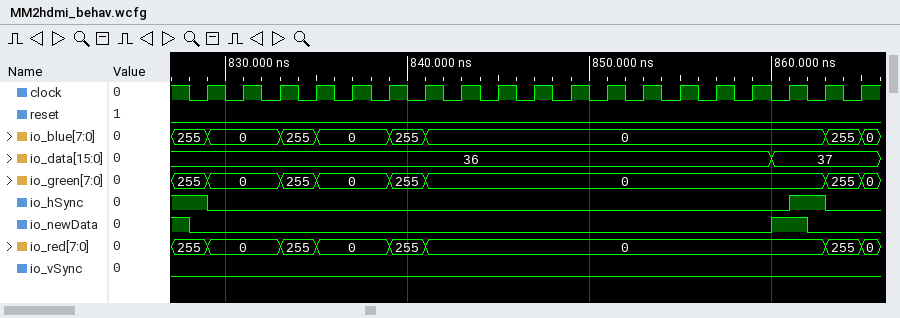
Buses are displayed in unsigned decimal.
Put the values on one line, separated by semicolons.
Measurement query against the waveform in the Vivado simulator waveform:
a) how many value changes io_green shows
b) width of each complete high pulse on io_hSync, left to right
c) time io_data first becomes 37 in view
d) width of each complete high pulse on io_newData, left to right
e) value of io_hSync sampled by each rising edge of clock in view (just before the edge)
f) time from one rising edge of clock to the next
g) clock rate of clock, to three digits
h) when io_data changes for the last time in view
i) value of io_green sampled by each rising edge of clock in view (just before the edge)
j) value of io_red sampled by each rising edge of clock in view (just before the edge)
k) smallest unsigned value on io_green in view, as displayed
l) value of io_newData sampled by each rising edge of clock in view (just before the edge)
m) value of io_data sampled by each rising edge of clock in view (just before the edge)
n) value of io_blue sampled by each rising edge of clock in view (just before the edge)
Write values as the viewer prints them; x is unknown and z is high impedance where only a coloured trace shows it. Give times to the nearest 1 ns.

7; 2 ns; 860 ns; 2 ns; 1 0 0 0 0 0 0 0 0 0 0 0 0 0 0 0 0 1 0; 2 ns; 500 MHz; 860 ns; 255, 0, 0, 255, 0, 0, 255, 0, 0, 0, 0, 0, 0, 0, 0, 0, 0, 0, 255; 255, 0, 0, 255, 0, 0, 255, 0, 0, 0, 0, 0, 0, 0, 0, 0, 0, 0, 255; 0; 0 0 0 0 0 0 0 0 0 0 0 0 0 0 0 0 1 0 0; 36, 36, 36, 36, 36, 36, 36, 36, 36, 36, 36, 36, 36, 36, 36, 36, 37, 37, 37; 255, 0, 0, 255, 0, 0, 255, 0, 0, 0, 0, 0, 0, 0, 0, 0, 0, 0, 255
